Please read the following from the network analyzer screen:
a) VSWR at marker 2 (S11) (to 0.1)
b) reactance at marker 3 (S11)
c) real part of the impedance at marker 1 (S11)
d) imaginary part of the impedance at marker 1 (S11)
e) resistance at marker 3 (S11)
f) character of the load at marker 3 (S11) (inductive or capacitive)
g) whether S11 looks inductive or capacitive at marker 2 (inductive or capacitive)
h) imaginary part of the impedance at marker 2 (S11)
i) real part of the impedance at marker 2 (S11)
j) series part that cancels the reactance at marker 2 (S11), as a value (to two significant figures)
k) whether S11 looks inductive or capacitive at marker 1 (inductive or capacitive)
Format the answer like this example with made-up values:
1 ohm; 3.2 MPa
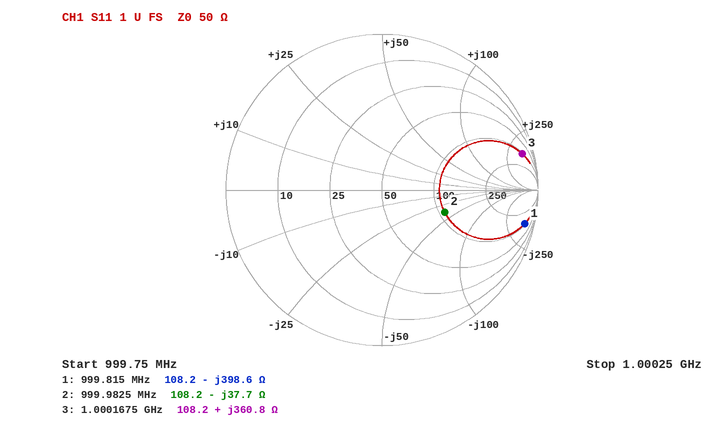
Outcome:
2.5; +360.8 Ω; 108.2 Ω; -398.6 Ω; 108.2 Ω; inductive; capacitive; -37.7 Ω; 108.2 Ω; 6.0 nH; capacitive
